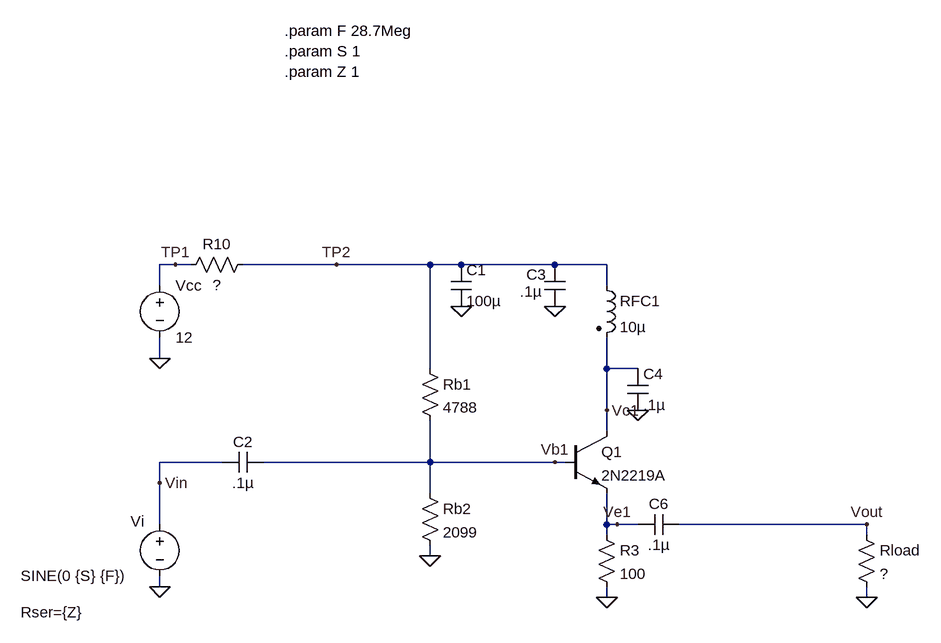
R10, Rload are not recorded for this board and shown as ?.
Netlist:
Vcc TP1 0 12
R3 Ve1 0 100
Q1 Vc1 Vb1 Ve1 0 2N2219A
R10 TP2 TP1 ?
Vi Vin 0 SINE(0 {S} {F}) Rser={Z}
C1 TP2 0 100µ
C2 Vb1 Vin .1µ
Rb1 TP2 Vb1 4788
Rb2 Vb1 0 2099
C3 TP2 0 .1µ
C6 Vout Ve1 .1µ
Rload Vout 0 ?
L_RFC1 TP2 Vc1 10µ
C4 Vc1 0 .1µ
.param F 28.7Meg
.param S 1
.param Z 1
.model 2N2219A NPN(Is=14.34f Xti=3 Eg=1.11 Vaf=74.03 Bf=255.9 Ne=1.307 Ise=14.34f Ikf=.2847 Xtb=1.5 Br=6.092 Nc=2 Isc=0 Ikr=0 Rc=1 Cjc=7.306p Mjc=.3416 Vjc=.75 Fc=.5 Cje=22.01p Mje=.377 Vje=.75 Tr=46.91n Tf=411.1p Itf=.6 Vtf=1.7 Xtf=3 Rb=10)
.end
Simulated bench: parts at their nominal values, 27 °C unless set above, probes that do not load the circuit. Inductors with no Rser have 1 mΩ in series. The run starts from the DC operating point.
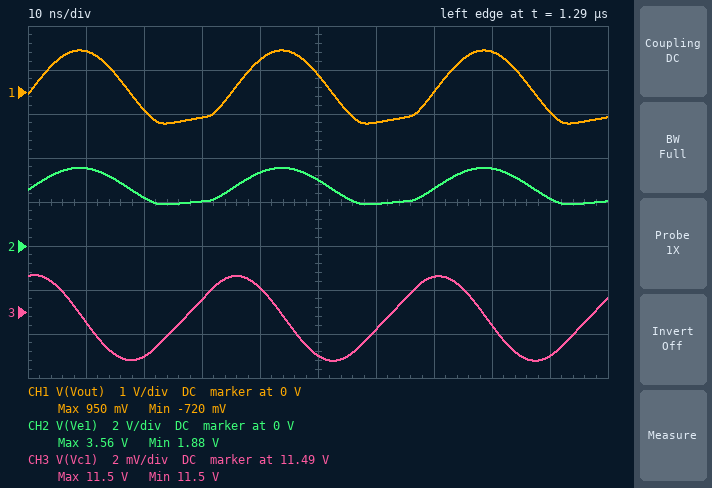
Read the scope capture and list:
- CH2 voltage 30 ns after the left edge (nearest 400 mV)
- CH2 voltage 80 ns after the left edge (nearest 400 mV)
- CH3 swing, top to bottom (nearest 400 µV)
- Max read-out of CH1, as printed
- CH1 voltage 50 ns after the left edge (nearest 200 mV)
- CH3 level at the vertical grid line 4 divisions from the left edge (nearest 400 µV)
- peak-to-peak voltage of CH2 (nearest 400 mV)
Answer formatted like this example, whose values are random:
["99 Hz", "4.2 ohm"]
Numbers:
["2.0 V", "3.6 V", "4.0 mV", "950 mV", "400 mV", "11.4872 V", "1.6 V"]
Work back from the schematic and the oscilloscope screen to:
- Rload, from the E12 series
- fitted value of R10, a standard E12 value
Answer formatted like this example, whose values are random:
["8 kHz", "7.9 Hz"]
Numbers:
["33 Ω", "18 Ω"]
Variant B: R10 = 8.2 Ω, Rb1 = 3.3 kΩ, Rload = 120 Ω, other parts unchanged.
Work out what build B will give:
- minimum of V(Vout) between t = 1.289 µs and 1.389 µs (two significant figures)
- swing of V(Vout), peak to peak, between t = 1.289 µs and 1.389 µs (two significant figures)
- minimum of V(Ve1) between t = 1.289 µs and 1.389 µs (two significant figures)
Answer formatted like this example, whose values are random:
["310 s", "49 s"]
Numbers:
["-980 mV", "2.0 V", "2.6 V"]
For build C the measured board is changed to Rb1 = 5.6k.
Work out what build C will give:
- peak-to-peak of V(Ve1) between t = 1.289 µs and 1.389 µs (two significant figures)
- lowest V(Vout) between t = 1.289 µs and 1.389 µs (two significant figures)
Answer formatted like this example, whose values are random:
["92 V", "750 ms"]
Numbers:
["1.6 V", "-650 mV"]
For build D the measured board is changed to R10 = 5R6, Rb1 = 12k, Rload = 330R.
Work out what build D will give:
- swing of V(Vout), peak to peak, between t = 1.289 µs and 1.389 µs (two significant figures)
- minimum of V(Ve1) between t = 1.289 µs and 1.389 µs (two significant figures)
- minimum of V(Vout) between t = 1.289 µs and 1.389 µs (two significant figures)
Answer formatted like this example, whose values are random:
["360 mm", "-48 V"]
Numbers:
["1.8 V", "140 mV", "-850 mV"]
